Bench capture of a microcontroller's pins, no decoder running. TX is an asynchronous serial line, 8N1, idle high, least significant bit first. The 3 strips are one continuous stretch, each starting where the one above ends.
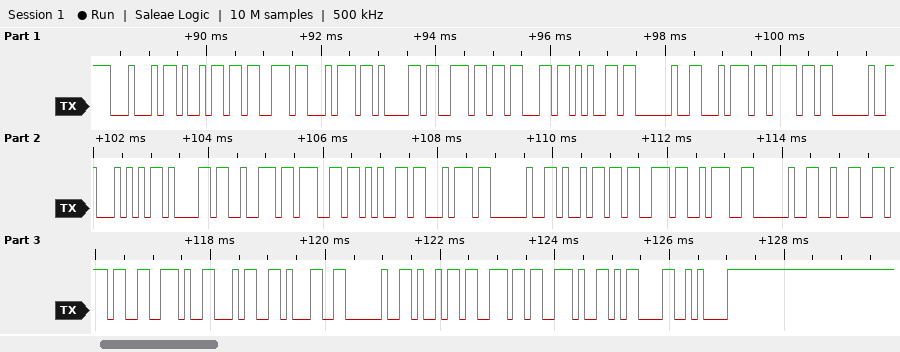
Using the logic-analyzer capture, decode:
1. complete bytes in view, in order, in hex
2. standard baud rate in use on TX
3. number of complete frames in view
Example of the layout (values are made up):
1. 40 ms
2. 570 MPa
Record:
1. 0x44 0x69 0x73 0x74 0x61 0x6E 0x63 0x65 0x20 0x74 0x6F 0x20 0x54 0x61 0x72 0x67 0x65 0x74 0x20 0x69 0x73 0x3A 0x20 0x32 0x37 0x2E 0x34 0x31 0x20 0x69 0x6E 0x2E 0x0D 0x0A
2. 9600 baud
3. 34
